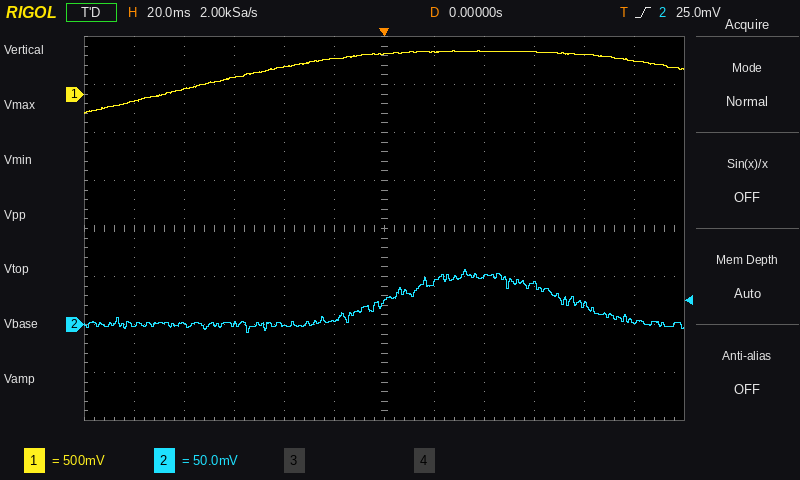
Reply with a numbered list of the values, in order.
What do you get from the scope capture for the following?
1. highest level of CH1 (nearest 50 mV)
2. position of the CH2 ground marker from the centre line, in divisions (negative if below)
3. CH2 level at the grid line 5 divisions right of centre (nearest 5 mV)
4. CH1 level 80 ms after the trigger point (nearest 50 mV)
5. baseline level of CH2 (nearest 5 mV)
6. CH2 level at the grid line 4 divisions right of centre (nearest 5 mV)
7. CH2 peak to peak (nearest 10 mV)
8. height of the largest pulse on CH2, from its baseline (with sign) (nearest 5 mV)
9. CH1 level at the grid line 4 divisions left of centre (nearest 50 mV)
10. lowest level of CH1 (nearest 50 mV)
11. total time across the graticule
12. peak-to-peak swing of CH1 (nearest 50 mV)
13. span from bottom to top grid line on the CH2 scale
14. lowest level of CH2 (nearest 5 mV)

1. 450 mV
2. -2.0 div
3. 5 mV
4. 400 mV
5. 0 mV
6. 20 mV
7. 70 mV
8. +55 mV
9. 50 mV
10. -200 mV
11. 240 ms
12. 650 mV
13. 400 mV
14. -10 mV
